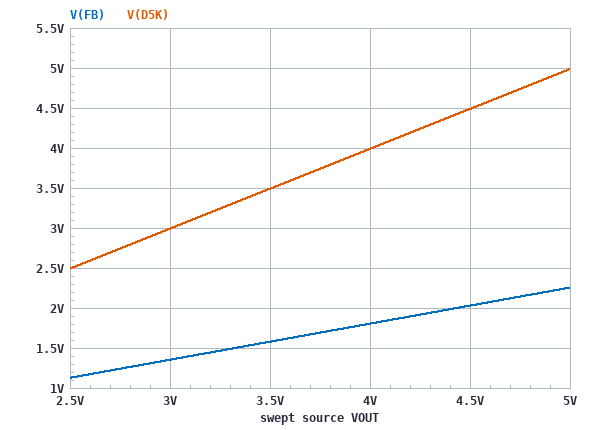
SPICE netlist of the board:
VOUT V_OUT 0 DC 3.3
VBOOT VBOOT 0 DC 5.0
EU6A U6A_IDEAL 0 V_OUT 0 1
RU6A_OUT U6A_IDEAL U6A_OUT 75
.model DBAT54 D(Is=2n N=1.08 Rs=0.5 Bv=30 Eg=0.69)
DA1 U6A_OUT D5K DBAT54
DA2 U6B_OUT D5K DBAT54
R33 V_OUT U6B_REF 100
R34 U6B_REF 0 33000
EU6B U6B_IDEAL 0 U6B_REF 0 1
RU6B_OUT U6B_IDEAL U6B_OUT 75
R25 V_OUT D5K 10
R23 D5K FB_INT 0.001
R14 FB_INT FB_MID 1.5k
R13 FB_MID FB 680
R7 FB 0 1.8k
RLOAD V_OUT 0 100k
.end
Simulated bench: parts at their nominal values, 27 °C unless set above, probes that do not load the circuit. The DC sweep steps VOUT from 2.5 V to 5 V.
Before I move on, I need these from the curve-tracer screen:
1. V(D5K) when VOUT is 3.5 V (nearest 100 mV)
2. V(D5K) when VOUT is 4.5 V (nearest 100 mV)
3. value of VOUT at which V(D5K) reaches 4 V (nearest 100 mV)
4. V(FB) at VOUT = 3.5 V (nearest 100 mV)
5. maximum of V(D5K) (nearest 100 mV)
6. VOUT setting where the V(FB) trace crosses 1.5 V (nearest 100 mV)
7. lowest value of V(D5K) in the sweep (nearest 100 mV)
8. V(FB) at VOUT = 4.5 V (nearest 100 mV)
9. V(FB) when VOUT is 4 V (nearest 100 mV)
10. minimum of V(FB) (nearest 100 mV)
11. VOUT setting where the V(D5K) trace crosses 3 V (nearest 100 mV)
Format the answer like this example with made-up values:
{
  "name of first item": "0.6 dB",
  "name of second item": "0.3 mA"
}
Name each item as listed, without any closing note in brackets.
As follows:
{
  "V(D5K) when VOUT is 3.5 V": "3.5 V",
  "V(D5K) when VOUT is 4.5 V": "4.5 V",
  "value of VOUT at which V(D5K) reaches 4 V": "4.0 V",
  "V(FB) at VOUT = 3.5 V": "1.6 V",
  "maximum of V(D5K)": "5.0 V",
  "VOUT setting where the V(FB) trace crosses 1.5 V": "3.3 V",
  "lowest value of V(D5K) in the sweep": "2.5 V",
  "V(FB) at VOUT = 4.5 V": "2.0 V",
  "V(FB) when VOUT is 4 V": "1.8 V",
  "minimum of V(FB)": "1.1 V",
  "VOUT setting where the V(D5K) trace crosses 3 V": "3.0 V"
}
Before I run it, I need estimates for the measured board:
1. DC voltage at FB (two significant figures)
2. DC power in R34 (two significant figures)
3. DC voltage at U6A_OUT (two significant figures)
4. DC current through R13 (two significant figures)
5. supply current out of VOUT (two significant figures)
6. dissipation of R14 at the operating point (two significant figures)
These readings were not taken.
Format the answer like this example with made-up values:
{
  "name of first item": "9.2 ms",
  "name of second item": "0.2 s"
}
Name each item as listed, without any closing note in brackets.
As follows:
{
  "DC voltage at FB": "1.5 V",
  "DC power in R34": "330 µW",
  "DC voltage at U6A_OUT": "3.3 V",
  "DC current through R13": "830 µA",
  "supply current out of VOUT": "960 µA",
  "dissipation of R14 at the operating point": "1.0 mW"
}
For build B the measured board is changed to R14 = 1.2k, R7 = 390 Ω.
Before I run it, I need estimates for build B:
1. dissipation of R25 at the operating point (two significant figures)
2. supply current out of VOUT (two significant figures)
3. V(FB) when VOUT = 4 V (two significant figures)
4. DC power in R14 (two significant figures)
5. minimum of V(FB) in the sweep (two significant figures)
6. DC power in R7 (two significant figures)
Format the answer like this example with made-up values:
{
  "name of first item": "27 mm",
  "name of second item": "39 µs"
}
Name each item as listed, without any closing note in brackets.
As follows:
{
  "dissipation of R25 at the operating point": "21 µW",
  "supply current out of VOUT": "1.6 mA",
  "V(FB) when VOUT = 4 V": "680 mV",
  "DC power in R14": "2.5 mW",
  "minimum of V(FB) in the sweep": "430 mV",
  "DC power in R7": "820 µW"
}
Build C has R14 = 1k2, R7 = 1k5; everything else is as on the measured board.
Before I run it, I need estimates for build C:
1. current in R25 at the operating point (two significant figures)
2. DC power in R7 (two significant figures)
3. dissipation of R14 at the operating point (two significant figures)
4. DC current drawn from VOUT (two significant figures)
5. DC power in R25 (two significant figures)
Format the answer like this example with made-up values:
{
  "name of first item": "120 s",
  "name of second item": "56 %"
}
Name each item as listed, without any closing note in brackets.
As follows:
{
  "current in R25 at the operating point": "970 µA",
  "DC power in R7": "1.4 mW",
  "dissipation of R14 at the operating point": "1.1 mW",
  "DC current drawn from VOUT": "1.1 mA",
  "DC power in R25": "9.5 µW"
}
